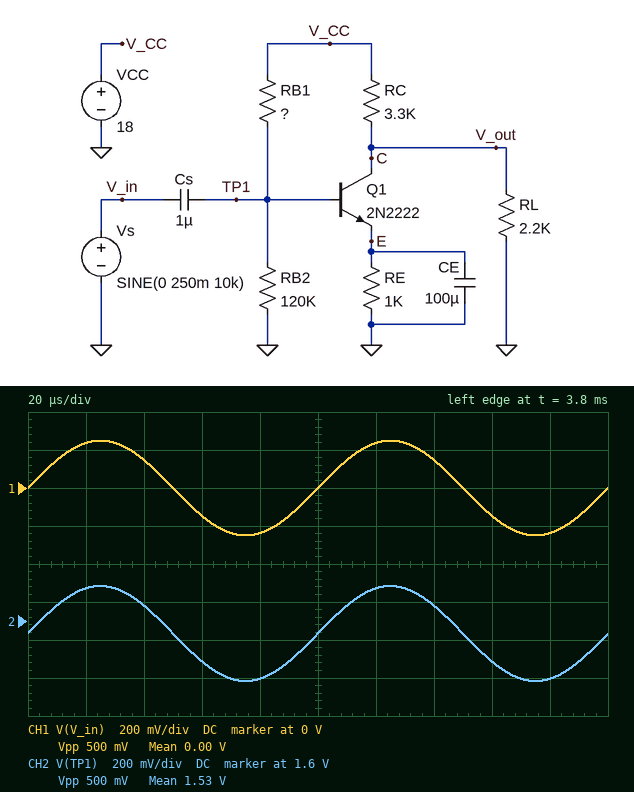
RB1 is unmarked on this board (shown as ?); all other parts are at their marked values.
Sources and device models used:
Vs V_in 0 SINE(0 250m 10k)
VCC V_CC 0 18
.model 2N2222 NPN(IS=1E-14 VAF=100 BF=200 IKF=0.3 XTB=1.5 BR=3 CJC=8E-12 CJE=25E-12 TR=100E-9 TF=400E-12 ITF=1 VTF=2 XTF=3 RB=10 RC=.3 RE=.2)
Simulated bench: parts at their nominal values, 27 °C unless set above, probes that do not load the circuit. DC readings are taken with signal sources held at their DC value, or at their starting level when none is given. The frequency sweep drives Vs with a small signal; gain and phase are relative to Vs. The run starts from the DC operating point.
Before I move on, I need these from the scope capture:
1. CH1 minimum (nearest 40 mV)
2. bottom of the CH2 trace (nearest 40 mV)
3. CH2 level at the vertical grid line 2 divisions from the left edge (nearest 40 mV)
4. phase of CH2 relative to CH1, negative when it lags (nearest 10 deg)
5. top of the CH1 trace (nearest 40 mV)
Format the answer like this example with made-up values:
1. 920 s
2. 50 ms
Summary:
1. -240 mV
2. 1.28 V
3. 1.68 V
4. 0 deg
5. 240 mV
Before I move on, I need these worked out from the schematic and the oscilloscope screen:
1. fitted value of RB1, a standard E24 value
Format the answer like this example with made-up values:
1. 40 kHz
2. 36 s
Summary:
1. 820 kΩ
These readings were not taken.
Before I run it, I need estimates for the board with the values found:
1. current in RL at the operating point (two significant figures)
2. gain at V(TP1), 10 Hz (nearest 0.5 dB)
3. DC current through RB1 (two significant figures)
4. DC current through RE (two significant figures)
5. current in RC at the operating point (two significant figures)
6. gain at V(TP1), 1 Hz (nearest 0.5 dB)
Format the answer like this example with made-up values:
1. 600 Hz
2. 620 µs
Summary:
1. 2.6 mA
2. -3.5 dB
3. 20 µA
4. 1.1 mA
5. 3.7 mA
6. -8.5 dB
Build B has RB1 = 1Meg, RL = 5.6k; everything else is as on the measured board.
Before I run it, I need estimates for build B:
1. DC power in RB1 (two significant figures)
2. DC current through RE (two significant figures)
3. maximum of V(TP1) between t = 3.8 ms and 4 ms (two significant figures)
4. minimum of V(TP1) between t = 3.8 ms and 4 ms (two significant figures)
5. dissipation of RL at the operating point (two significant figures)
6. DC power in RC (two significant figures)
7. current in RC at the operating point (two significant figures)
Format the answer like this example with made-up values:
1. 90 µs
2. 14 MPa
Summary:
1. 270 µW
2. 860 µA
3. 1.6 V
4. 1.1 V
5. 16 mW
6. 22 mW
7. 2.6 mA
